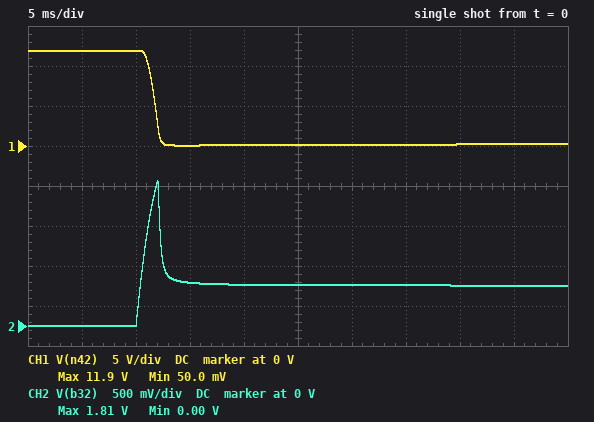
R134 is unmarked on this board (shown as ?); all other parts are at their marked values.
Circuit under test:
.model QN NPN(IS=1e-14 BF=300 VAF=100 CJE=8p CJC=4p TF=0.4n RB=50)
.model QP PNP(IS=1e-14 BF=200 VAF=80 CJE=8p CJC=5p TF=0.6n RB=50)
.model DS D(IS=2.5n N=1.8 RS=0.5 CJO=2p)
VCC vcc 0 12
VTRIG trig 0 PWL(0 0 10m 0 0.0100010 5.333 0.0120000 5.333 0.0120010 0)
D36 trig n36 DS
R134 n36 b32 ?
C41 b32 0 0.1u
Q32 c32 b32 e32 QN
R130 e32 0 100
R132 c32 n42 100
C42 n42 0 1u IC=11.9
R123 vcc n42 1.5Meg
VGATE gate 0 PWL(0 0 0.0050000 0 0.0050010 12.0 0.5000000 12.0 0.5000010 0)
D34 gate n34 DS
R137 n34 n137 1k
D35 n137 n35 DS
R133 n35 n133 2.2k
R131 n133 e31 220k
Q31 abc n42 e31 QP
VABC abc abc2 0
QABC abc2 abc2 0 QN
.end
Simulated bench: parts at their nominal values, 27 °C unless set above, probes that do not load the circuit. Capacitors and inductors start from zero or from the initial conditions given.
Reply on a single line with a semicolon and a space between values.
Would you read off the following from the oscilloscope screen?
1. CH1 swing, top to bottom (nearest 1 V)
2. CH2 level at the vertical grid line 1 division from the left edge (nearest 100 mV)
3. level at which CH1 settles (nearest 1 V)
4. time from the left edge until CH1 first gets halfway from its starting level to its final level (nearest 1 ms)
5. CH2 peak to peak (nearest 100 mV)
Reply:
12 V; 0 V; 0 V; 12 ms; 1.8 V
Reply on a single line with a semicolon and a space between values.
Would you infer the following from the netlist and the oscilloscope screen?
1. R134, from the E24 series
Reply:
36 kΩ
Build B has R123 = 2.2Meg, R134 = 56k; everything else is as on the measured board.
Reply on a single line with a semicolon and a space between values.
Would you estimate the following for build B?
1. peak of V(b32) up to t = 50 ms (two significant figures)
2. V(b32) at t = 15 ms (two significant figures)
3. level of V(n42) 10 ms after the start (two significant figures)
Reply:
1.3 V; 560 mV; 12 V
